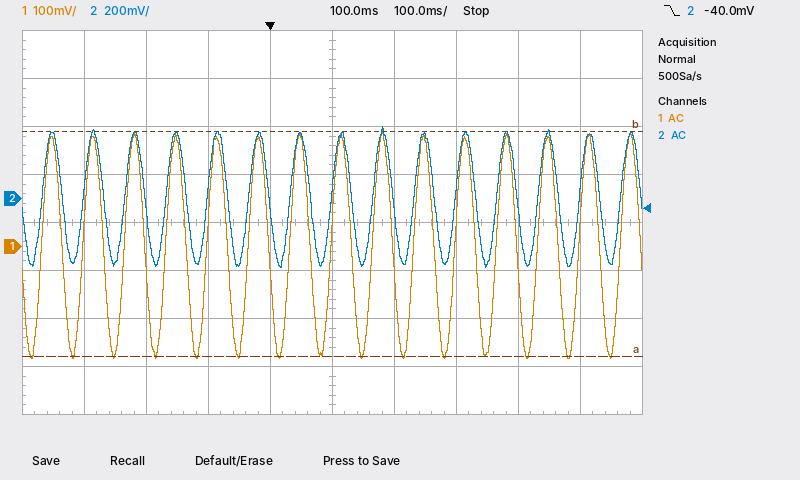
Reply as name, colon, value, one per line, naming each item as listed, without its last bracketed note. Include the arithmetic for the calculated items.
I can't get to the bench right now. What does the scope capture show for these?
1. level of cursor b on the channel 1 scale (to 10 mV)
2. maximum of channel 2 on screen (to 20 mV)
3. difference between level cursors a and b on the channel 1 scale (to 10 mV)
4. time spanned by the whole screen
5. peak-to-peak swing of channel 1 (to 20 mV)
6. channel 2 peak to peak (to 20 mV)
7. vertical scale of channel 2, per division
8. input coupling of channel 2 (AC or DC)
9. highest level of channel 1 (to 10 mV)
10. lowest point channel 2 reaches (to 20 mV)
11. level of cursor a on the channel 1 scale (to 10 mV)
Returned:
level of cursor b on the channel 1 scale: 240 mV
maximum of channel 2 on screen: 300 mV
difference between level cursors a and b on the channel 1 scale: 470 mV
time spanned by the whole screen: 1 s
peak-to-peak swing of channel 1: 480 mV
channel 2 peak to peak: 300 mV − (-280 mV) = 580 mV
vertical scale of channel 2, per division: 200 mV
input coupling of channel 2: AC
highest level of channel 1: 240 mV
lowest point channel 2 reaches: -280 mV
level of cursor a on the channel 1 scale: -230 mV
